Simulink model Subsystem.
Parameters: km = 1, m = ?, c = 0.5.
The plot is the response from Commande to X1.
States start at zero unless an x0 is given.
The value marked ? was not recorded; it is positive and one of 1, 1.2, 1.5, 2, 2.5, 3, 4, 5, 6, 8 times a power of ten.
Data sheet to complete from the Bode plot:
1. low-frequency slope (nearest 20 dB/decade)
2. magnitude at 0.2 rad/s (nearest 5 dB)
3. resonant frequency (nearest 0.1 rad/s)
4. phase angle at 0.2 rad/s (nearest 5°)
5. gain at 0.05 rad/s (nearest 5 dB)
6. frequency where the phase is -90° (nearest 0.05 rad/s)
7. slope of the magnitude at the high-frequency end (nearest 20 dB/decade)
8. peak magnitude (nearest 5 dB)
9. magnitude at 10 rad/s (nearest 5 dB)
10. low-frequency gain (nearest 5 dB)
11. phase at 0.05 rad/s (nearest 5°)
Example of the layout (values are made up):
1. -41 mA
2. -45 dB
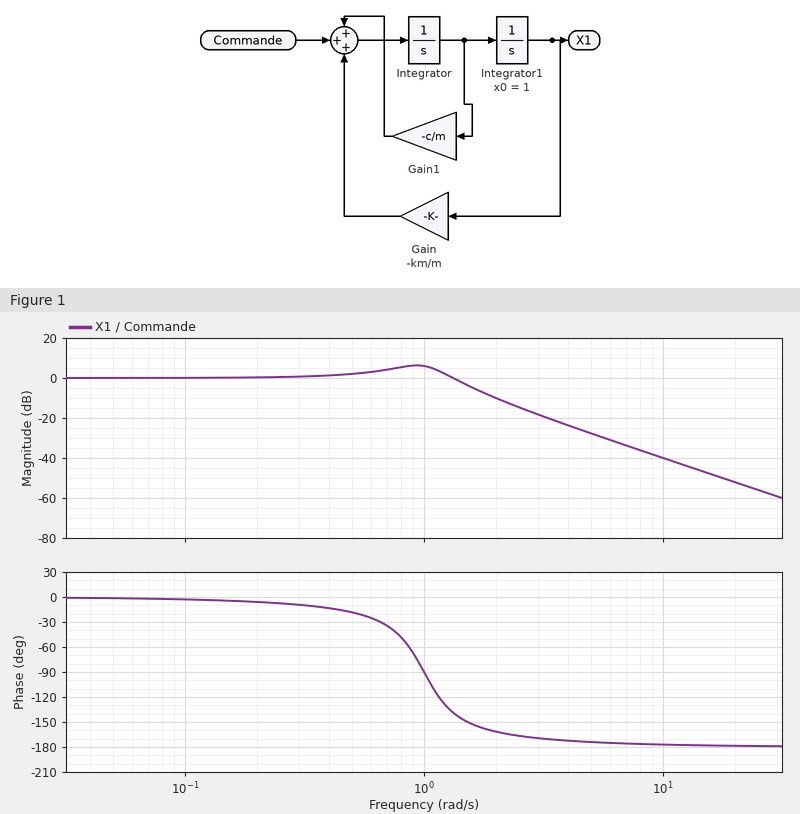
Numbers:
1. 0 dB/decade
2. 0 dB
3. 0.9 rad/s
4. -5°
5. 0 dB
6. 1.00 rad/s
7. -40 dB/decade
8. 5 dB
9. -40 dB
10. 0 dB
11. 0°
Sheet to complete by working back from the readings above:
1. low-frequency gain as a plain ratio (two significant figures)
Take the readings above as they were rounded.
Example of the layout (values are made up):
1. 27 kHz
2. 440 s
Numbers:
1. 1.0
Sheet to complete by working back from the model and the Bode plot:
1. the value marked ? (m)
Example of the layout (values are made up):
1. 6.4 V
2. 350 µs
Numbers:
1. 1
